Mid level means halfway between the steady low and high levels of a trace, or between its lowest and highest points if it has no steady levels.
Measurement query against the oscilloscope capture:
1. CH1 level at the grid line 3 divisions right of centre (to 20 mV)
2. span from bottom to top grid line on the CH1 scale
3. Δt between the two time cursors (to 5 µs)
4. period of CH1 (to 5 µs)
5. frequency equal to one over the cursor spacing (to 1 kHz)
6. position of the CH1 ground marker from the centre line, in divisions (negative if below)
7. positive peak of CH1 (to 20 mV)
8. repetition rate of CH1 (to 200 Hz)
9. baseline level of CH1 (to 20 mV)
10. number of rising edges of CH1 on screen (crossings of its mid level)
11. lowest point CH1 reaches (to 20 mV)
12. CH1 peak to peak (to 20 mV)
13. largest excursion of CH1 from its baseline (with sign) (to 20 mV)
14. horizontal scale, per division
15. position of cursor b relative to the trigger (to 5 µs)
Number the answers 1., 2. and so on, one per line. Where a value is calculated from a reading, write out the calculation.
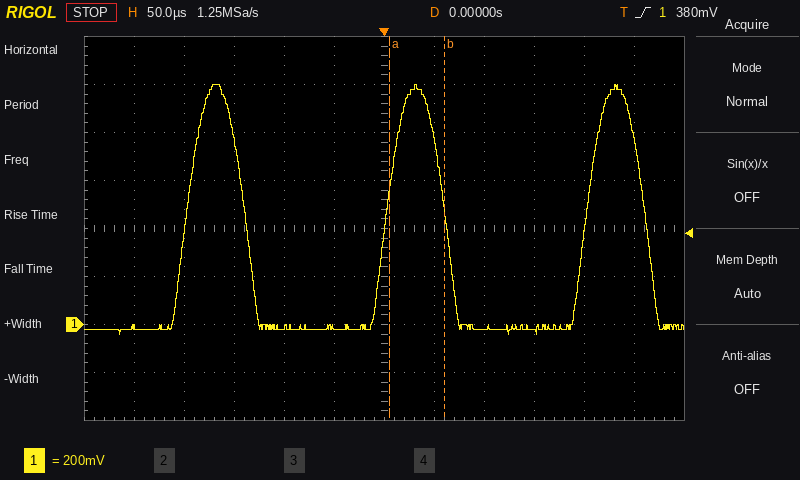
1. -20 mV
2. 1.6 V
3. 55 µs
4. 200 µs
5. 1 / 55 µs ≈ 18 kHz
6. -2.0 div
7. 1.00 V
8. 1 / 200 µs ≈ 5.0 kHz
9. -20 mV
10. 3
11. -40 mV
12. 1.00 V − (-40 mV) = 1.04 V
13. 1.00 V − (-20 mV) = +1.02 V
14. 50 µs
15. +60 µs
